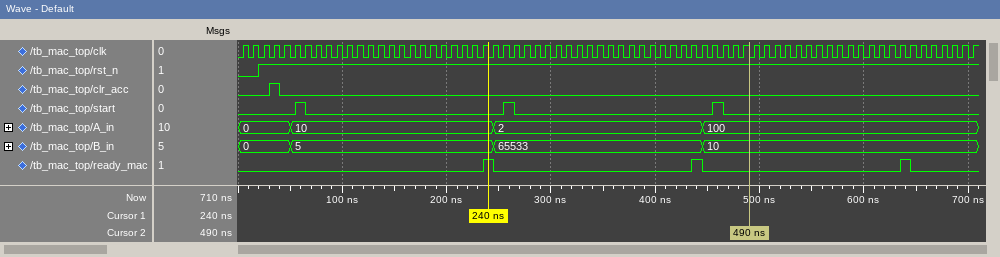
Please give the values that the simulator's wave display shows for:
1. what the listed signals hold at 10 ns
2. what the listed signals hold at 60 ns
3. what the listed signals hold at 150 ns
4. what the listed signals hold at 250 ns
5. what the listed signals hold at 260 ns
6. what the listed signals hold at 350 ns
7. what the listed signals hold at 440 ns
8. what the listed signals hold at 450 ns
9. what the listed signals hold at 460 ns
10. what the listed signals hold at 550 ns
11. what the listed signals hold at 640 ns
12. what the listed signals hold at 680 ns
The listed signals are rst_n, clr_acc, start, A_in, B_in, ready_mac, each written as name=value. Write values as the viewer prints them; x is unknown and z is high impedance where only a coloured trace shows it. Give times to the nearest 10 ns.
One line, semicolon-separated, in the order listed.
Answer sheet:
rst_n=0, clr_acc=0, start=0, A_in=0, B_in=0, ready_mac=0; rst_n=1, clr_acc=0, start=1, A_in=10, B_in=5, ready_mac=0; rst_n=1, clr_acc=0, start=0, A_in=10, B_in=5, ready_mac=0; rst_n=1, clr_acc=0, start=0, A_in=2, B_in=65533, ready_mac=0; rst_n=1, clr_acc=0, start=1, A_in=2, B_in=65533, ready_mac=0; rst_n=1, clr_acc=0, start=0, A_in=2, B_in=65533, ready_mac=0; rst_n=1, clr_acc=0, start=0, A_in=2, B_in=65533, ready_mac=1; rst_n=1, clr_acc=0, start=0, A_in=100, B_in=10, ready_mac=0; rst_n=1, clr_acc=0, start=1, A_in=100, B_in=10, ready_mac=0; rst_n=1, clr_acc=0, start=0, A_in=100, B_in=10, ready_mac=0; rst_n=1, clr_acc=0, start=0, A_in=100, B_in=10, ready_mac=1; rst_n=1, clr_acc=0, start=0, A_in=100, B_in=10, ready_mac=0
